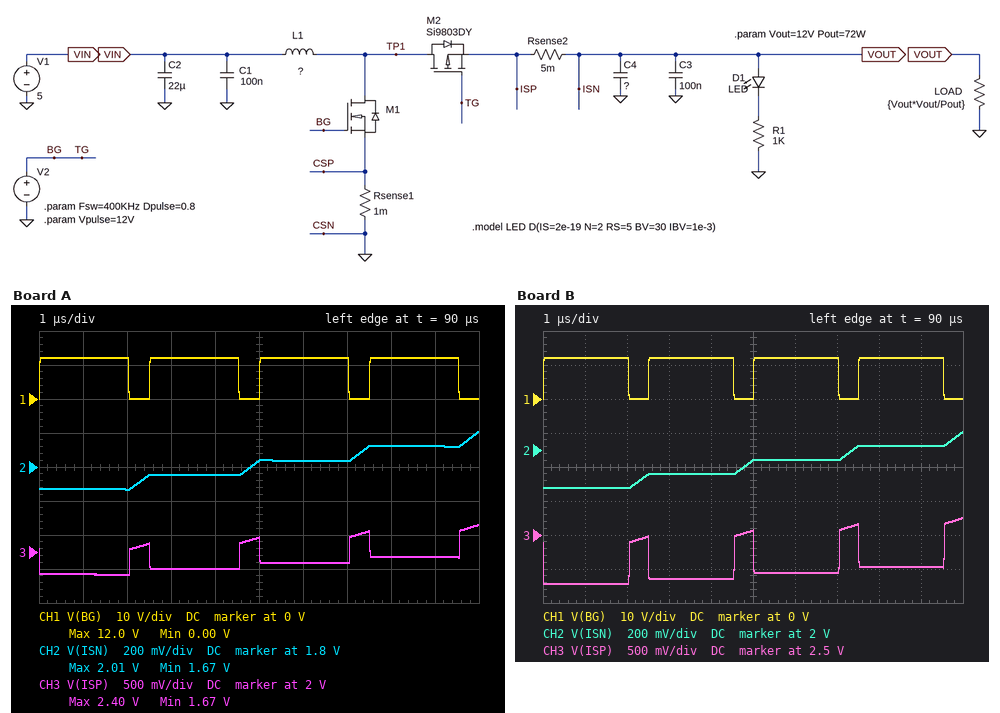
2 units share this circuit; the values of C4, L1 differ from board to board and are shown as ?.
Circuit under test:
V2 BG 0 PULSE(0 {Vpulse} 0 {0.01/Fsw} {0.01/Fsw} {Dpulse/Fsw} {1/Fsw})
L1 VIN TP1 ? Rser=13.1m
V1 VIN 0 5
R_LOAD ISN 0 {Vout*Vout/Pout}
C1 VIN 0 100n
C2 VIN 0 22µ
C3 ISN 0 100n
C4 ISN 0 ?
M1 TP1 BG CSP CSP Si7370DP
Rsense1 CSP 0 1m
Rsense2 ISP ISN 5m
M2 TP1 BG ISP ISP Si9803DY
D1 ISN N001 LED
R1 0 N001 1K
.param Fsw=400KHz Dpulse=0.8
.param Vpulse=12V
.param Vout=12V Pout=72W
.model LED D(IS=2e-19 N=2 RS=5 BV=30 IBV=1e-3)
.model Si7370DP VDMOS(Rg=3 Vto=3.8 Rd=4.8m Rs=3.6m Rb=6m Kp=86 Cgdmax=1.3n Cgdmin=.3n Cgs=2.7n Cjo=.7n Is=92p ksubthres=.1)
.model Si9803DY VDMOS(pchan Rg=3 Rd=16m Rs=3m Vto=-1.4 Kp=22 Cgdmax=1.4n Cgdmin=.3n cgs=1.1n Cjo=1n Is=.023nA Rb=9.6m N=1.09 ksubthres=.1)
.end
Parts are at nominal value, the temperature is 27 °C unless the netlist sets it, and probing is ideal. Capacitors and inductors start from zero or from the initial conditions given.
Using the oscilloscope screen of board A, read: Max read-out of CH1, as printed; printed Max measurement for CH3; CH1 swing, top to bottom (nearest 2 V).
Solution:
12.0 V
2.40 V
12 V
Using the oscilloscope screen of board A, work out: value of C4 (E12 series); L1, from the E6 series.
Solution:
390 µF
4.7 µH
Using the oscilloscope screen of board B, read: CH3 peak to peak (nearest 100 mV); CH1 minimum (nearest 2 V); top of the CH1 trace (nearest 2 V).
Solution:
1.0 V
0 V
12 V
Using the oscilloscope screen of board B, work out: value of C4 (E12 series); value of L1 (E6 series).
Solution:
680 µF
2.2 µH
